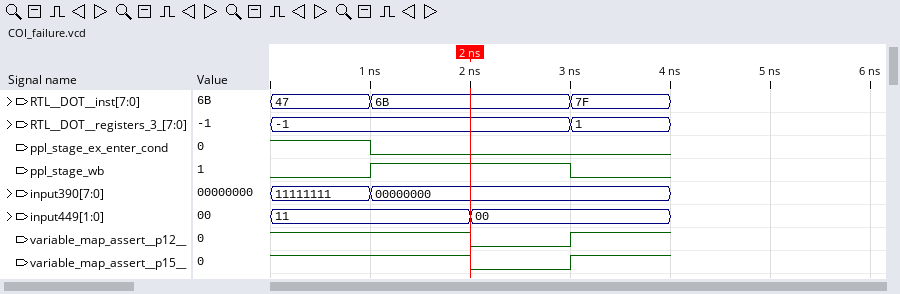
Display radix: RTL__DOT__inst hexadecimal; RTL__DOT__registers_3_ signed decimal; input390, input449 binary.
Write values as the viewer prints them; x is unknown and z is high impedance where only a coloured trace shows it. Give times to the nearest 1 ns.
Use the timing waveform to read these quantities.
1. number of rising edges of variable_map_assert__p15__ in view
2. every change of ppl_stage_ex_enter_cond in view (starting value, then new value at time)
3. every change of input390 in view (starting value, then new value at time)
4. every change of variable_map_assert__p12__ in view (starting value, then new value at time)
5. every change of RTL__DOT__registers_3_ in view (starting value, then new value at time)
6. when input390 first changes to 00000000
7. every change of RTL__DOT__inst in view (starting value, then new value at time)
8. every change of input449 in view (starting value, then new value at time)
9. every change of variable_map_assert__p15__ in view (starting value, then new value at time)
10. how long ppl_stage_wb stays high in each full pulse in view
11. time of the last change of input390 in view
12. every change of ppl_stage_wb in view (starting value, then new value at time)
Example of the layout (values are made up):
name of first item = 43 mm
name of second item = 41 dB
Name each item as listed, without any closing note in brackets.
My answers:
number of rising edges of variable_map_assert__p15__ in view = 1
every change of ppl_stage_ex_enter_cond in view = 1, 0 at 1 ns
every change of input390 in view = 11111111, 00000000 at 1 ns
every change of variable_map_assert__p12__ in view = 1, 0 at 2 ns, 1 at 3 ns
every change of RTL__DOT__registers_3_ in view = -1, 1 at 3 ns
when input390 first changes to 00000000 = 1 ns
every change of RTL__DOT__inst in view = 47, 6B at 1 ns, 7F at 3 ns
every change of input449 in view = 11, 00 at 2 ns
every change of variable_map_assert__p15__ in view = 1, 0 at 2 ns, 1 at 3 ns
how long ppl_stage_wb stays high in each full pulse in view = 2 ns
time of the last change of input390 in view = 1 ns
every change of ppl_stage_wb in view = 0, 1 at 1 ns, 0 at 3 ns
